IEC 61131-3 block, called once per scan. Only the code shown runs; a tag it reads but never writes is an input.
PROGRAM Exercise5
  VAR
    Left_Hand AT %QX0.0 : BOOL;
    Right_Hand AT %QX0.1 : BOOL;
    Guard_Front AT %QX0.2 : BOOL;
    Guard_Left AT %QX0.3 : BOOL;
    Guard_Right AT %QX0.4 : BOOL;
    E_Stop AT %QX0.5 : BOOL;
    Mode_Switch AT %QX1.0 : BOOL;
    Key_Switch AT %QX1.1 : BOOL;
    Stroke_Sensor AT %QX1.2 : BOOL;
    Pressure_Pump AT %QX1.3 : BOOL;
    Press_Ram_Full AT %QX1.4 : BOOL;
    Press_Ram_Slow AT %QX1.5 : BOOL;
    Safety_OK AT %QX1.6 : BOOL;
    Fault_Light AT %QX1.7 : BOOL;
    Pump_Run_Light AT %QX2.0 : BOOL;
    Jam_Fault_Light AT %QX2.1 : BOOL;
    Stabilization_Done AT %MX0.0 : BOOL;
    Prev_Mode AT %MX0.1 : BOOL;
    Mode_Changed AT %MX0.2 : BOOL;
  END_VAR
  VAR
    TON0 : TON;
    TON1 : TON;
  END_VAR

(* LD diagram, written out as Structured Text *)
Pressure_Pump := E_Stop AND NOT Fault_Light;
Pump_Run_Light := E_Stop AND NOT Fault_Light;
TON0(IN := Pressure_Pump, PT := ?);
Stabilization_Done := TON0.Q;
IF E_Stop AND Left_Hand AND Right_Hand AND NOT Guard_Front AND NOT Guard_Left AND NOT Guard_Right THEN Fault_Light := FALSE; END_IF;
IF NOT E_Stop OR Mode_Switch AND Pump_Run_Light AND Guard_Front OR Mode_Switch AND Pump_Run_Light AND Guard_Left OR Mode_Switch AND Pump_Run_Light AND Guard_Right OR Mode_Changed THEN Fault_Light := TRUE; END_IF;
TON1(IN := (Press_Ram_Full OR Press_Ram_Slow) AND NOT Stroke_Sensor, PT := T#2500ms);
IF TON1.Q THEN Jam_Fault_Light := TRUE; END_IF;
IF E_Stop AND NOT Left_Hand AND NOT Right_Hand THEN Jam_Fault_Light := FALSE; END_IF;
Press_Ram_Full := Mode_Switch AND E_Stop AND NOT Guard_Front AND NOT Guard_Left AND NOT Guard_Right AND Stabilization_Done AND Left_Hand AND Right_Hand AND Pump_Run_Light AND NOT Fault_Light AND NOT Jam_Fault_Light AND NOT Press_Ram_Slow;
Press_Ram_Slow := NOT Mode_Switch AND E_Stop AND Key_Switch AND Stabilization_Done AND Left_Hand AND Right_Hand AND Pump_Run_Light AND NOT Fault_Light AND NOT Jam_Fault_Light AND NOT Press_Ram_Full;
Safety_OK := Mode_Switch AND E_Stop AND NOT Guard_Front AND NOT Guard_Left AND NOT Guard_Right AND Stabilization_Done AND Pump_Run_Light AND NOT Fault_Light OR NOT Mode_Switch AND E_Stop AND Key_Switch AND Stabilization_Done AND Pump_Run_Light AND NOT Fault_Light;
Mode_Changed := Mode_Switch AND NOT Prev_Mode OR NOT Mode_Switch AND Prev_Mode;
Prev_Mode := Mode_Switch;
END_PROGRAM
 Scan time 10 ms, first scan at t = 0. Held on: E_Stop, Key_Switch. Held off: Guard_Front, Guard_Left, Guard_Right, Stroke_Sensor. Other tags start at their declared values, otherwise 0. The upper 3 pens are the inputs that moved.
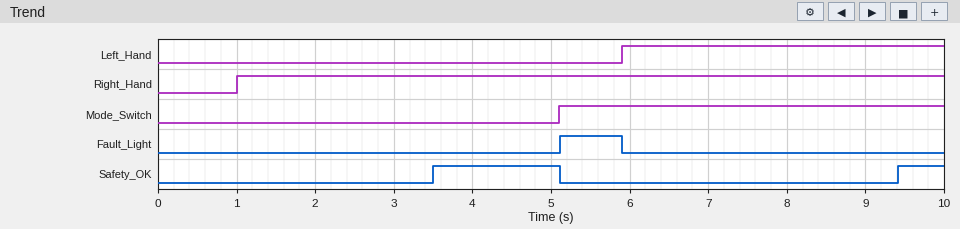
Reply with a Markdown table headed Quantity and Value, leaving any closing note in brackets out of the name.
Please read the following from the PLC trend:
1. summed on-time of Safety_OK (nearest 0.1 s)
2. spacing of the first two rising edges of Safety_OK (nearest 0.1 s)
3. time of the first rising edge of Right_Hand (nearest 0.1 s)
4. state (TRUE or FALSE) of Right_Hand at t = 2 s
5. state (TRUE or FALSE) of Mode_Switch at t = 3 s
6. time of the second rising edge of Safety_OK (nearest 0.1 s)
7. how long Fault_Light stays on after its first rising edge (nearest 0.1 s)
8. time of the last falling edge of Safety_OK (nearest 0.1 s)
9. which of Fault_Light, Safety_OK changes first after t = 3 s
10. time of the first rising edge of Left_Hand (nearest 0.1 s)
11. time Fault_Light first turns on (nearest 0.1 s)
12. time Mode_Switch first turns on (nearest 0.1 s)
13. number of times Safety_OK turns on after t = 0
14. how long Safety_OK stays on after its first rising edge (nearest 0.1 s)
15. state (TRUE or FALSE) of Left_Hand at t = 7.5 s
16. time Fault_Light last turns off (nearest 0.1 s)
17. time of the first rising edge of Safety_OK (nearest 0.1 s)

| Quantity | Value |
|---|---|
| summed on-time of Safety_OK | 2.2 s |
| spacing of the first two rising edges of Safety_OK | 5.9 s |
| time of the first rising edge of Right_Hand | 1.0 s |
| state (TRUE or FALSE) of Right_Hand at t = 2 s | TRUE |
| state (TRUE or FALSE) of Mode_Switch at t = 3 s | FALSE |
| time of the second rising edge of Safety_OK | 9.4 s |
| how long Fault_Light stays on after its first rising edge | 0.8 s |
| time of the last falling edge of Safety_OK | 5.1 s |
| which of Fault_Light, Safety_OK changes first after t = 3 s | Safety_OK |
| time of the first rising edge of Left_Hand | 5.9 s |
| time Fault_Light first turns on | 5.1 s |
| time Mode_Switch first turns on | 5.1 s |
| number of times Safety_OK turns on after t = 0 | 2 |
| how long Safety_OK stays on after its first rising edge | 1.6 s |
| state (TRUE or FALSE) of Left_Hand at t = 7.5 s | TRUE |
| time Fault_Light last turns off | 5.9 s |
| time of the first rising edge of Safety_OK | 3.5 s |
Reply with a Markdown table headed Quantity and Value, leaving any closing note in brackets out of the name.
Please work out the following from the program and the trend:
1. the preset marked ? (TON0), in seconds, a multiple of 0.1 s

| Quantity | Value |
|---|---|
| the preset marked ? (TON0), in seconds, a multiple of 0.1 s | 3.5 s |
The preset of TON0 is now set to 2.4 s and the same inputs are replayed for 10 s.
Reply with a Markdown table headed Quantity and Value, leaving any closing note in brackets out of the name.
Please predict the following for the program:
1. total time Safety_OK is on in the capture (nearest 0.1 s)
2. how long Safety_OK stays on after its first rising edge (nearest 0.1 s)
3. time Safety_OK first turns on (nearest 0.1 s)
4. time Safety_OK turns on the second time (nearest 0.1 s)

| Quantity | Value |
|---|---|
| total time Safety_OK is on in the capture | 4.4 s |
| how long Safety_OK stays on after its first rising edge | 2.7 s |
| time Safety_OK first turns on | 2.4 s |
| time Safety_OK turns on the second time | 8.3 s |
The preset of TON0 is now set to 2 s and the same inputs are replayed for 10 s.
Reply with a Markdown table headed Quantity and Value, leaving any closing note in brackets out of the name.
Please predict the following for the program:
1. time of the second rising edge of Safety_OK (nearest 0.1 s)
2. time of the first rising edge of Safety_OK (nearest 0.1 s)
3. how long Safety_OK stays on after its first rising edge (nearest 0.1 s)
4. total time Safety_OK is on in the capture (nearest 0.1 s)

| Quantity | Value |
|---|---|
| time of the second rising edge of Safety_OK | 7.9 s |
| time of the first rising edge of Safety_OK | 2.0 s |
| how long Safety_OK stays on after its first rising edge | 3.1 s |
| total time Safety_OK is on in the capture | 5.2 s |
